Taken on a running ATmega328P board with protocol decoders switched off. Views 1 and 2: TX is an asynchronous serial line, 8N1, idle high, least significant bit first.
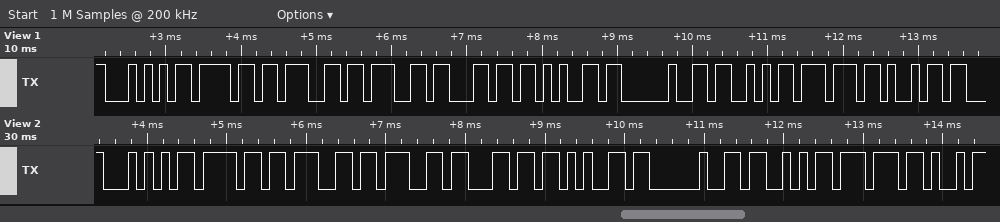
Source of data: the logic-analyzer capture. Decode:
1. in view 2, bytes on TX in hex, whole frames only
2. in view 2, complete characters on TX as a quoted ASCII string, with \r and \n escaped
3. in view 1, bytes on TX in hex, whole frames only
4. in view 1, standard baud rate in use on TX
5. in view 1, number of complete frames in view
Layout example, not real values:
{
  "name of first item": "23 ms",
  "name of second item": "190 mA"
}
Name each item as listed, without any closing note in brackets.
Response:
{
  "in view 2, bytes on TX in hex, whole frames only": "0x54 0x6F 0x67 0x67 0x6C 0x65 0x20 0x53 0x77",
  "in view 2, complete characters on TX as a quoted ASCII string, with \\r and \\n escaped": "\"Toggle Sw\"",
  "in view 1, bytes on TX in hex, whole frames only": "54 6F 67 67 6C 65 20 53 77 69",
  "in view 1, standard baud rate in use on TX": "9600 baud",
  "in view 1, number of complete frames in view": "10"
}
